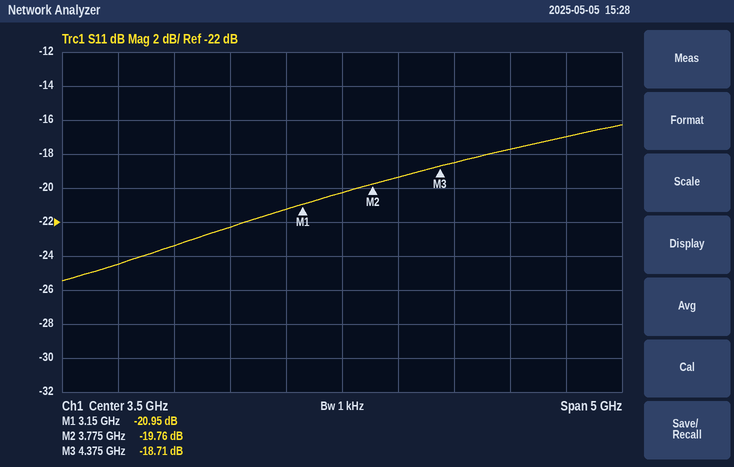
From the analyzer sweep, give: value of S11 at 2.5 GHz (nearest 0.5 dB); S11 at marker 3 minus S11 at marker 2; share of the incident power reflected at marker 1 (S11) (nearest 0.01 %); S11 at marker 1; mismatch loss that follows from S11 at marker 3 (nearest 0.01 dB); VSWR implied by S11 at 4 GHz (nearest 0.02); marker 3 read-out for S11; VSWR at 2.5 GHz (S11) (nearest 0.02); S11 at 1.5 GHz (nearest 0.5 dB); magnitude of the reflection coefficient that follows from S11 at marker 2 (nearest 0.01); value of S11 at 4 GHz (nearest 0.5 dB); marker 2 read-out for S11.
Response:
-22.5 dB
1.05 dB
0.80 %
-20.95 dB
0.06 dB
1.24
-18.71 dB
1.16
-24.5 dB
0.10
-19.5 dB
-19.76 dB
